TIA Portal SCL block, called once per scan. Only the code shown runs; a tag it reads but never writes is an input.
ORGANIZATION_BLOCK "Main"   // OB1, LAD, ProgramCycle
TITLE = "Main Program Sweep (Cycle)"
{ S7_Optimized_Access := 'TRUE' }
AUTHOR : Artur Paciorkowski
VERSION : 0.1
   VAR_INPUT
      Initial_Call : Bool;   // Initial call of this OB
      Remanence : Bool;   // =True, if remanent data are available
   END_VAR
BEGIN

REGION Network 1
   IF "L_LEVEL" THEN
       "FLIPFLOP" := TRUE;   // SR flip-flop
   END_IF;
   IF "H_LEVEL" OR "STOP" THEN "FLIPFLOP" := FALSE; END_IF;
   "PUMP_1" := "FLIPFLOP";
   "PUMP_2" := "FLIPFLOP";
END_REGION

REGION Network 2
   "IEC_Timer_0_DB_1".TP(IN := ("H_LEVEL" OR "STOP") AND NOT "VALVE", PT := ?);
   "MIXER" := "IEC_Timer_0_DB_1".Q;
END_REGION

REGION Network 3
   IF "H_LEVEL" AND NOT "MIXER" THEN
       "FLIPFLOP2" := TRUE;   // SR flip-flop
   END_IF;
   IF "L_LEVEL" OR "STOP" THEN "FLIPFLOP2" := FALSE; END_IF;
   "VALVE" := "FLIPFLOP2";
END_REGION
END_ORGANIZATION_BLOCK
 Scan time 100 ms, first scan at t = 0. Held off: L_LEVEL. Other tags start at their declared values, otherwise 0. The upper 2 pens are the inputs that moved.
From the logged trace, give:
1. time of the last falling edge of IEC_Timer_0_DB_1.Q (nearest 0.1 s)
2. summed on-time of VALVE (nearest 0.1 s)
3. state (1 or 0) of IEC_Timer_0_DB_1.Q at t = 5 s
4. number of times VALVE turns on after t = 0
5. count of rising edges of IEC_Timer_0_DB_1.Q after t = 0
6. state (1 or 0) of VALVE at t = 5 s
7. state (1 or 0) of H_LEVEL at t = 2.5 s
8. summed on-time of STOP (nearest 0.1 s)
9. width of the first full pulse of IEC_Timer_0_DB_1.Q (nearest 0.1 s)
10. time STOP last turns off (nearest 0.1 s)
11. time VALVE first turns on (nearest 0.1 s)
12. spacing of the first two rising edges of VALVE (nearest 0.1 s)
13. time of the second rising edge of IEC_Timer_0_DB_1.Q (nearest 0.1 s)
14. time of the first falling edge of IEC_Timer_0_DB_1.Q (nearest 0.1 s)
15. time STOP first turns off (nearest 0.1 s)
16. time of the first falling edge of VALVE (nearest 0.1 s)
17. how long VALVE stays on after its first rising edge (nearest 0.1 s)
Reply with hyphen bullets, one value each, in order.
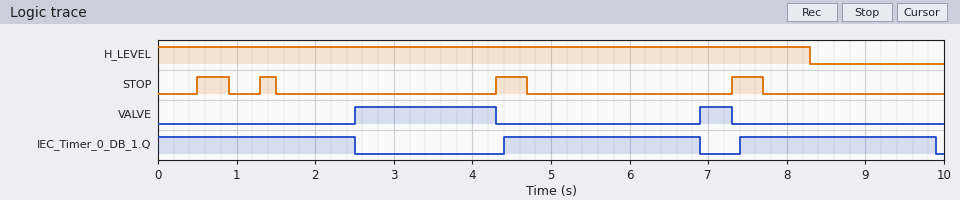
- 9.9 s
- 2.2 s
- 1
- 2
- 2
- 0
- 1
- 1.4 s
- 2.5 s
- 7.7 s
- 2.5 s
- 4.4 s
- 7.4 s
- 2.5 s
- 0.9 s
- 4.3 s
- 1.8 s
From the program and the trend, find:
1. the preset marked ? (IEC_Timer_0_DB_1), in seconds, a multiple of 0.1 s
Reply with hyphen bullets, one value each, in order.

- 2.5 s
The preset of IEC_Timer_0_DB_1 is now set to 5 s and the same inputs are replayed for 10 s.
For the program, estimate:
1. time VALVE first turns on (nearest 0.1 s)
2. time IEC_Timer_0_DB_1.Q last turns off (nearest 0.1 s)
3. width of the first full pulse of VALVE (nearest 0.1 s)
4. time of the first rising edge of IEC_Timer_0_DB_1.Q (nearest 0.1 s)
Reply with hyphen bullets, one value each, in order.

- 5.0 s
- 5.0 s
- 2.3 s
- 7.4 s
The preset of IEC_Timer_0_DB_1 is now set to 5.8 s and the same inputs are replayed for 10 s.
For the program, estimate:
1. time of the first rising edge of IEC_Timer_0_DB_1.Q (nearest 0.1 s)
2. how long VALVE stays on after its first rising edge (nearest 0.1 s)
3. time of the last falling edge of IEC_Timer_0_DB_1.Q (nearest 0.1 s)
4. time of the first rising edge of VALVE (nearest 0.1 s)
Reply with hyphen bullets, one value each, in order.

- 7.4 s
- 1.5 s
- 5.8 s
- 5.8 s
